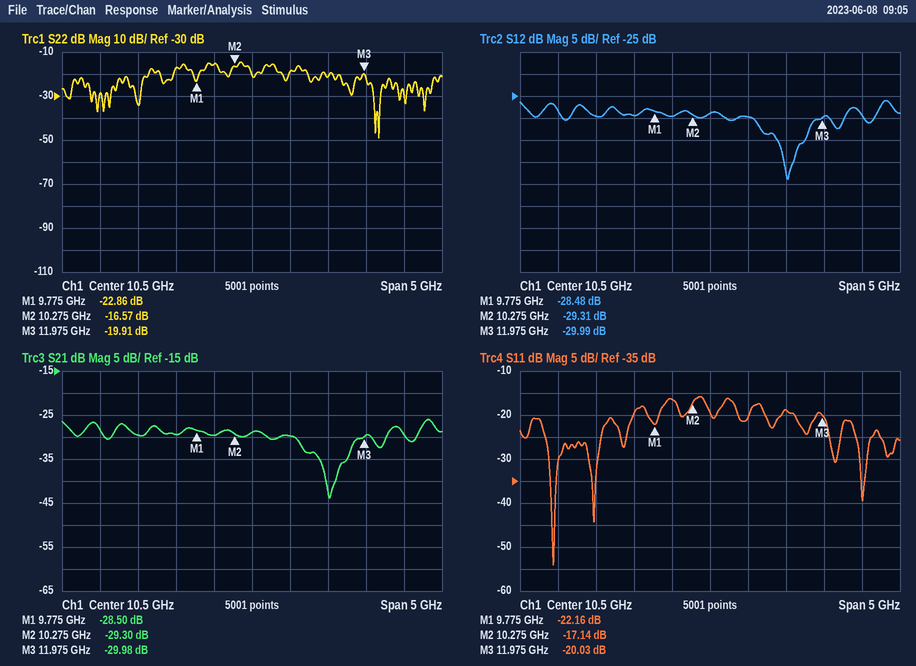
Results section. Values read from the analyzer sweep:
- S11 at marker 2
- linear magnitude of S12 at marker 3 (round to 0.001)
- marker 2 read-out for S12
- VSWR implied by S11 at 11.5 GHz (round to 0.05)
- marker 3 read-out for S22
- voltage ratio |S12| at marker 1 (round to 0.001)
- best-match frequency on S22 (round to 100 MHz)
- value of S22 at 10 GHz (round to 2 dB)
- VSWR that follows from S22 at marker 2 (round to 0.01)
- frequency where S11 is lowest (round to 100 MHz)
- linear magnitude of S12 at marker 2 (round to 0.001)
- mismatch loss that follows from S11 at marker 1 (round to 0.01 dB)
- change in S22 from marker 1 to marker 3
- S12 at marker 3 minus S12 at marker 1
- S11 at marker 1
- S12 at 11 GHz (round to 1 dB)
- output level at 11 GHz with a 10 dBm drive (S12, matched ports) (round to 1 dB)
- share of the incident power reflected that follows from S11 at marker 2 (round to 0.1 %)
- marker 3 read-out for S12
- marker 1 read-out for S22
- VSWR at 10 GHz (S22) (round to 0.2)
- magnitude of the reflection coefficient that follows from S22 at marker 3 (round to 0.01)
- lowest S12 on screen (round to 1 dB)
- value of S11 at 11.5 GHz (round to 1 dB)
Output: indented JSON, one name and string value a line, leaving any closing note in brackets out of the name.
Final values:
{
  "S11 at marker 2": "-17.14 dB",
  "linear magnitude of S12 at marker 3": "0.032",
  "marker 2 read-out for S12": "-29.31 dB",
  "VSWR implied by S11 at 11.5 GHz": "1.25",
  "marker 3 read-out for S22": "-19.91 dB",
  "voltage ratio |S12| at marker 1": "0.038",
  "best-match frequency on S22": "12.2 GHz",
  "value of S22 at 10 GHz": "-16 dB",
  "VSWR that follows from S22 at marker 2": "1.35",
  "frequency where S11 is lowest": "8.4 GHz",
  "linear magnitude of S12 at marker 2": "0.034",
  "mismatch loss that follows from S11 at marker 1": "0.03 dB",
  "change in S22 from marker 1 to marker 3": "2.95 dB",
  "S12 at marker 3 minus S12 at marker 1": "-1.51 dB",
  "S11 at marker 1": "-22.16 dB",
  "S12 at 11 GHz": "-30 dB",
  "output level at 11 GHz with a 10 dBm drive (S12, matched ports)": "-20 dBm",
  "share of the incident power reflected that follows from S11 at marker 2": "1.9 %",
  "marker 3 read-out for S12": "-29.99 dB",
  "marker 1 read-out for S22": "-22.86 dB",
  "VSWR at 10 GHz (S22)": "1.4",
  "magnitude of the reflection coefficient that follows from S22 at marker 3": "0.10",
  "lowest S12 on screen": "-44 dB",
  "value of S11 at 11.5 GHz": "-19 dB"
}
